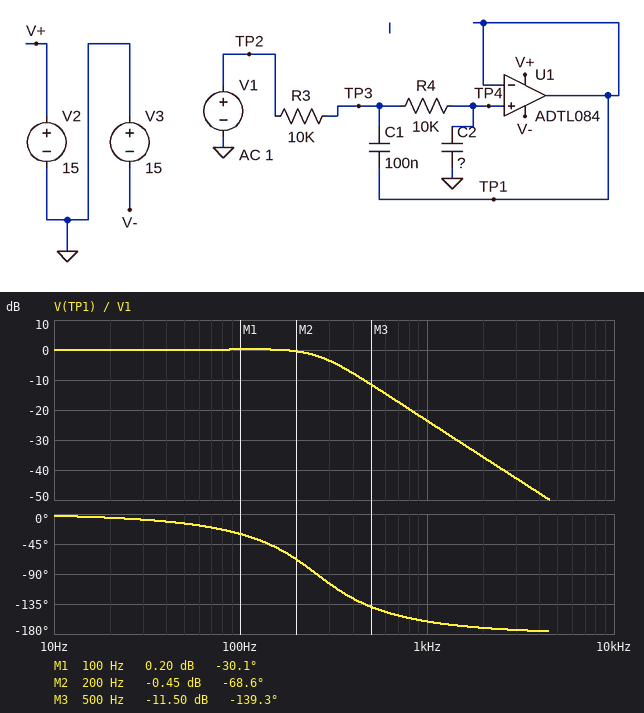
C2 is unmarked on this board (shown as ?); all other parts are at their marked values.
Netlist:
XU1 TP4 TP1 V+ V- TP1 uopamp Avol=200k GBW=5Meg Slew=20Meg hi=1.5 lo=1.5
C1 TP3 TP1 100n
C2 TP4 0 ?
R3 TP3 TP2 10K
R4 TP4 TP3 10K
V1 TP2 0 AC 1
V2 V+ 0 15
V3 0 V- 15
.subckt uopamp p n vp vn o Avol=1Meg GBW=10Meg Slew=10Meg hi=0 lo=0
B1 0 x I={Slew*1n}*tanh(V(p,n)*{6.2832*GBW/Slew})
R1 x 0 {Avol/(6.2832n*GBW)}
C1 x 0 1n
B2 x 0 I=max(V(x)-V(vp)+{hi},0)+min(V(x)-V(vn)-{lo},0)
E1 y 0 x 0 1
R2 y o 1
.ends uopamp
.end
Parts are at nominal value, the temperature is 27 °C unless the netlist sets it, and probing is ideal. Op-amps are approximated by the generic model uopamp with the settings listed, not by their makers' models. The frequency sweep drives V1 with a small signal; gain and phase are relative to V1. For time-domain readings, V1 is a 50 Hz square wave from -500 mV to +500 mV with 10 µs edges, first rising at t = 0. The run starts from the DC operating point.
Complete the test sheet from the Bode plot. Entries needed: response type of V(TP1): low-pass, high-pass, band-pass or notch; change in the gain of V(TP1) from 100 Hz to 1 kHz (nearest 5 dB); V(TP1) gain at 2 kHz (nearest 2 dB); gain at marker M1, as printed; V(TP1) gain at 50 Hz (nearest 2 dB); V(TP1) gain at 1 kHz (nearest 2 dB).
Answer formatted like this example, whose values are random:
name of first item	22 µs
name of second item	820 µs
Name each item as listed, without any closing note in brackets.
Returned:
response type of V(TP1): low-pass, high-pass, band-pass or notch	low-pass
change in the gain of V(TP1) from 100 Hz to 1 kHz	-25 dB
V(TP1) gain at 2 kHz	-36 dB
gain at marker M1, as printed	0.20 dB
V(TP1) gain at 50 Hz	0 dB
V(TP1) gain at 1 kHz	-24 dB
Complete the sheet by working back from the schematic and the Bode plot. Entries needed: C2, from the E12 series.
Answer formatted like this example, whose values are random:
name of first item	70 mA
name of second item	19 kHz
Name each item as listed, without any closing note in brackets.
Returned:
C2, from the E12 series	39 nF
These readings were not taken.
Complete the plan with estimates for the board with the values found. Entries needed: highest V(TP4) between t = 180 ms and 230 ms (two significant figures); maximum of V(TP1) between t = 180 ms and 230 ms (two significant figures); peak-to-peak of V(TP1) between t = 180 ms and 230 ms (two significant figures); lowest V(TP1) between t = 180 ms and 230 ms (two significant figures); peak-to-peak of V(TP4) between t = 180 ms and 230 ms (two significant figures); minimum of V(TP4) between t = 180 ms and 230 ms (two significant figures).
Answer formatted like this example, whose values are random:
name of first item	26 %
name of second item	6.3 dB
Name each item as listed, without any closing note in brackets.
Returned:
highest V(TP4) between t = 180 ms and 230 ms	580 mV
maximum of V(TP1) between t = 180 ms and 230 ms	580 mV
peak-to-peak of V(TP1) between t = 180 ms and 230 ms	1.2 V
lowest V(TP1) between t = 180 ms and 230 ms	-580 mV
peak-to-peak of V(TP4) between t = 180 ms and 230 ms	1.2 V
minimum of V(TP4) between t = 180 ms and 230 ms	-580 mV
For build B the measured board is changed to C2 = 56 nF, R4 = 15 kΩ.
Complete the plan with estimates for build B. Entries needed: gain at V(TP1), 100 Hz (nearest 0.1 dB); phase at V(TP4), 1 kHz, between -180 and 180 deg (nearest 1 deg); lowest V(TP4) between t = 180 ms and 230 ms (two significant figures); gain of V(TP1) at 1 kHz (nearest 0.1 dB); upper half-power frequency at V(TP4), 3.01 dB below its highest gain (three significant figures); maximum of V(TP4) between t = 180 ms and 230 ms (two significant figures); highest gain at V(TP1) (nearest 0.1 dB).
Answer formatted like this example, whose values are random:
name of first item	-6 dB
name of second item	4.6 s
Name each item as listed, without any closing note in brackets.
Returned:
gain at V(TP1), 100 Hz	-0.9 dB
phase at V(TP4), 1 kHz, between -180 and 180 deg	-165 deg
lowest V(TP4) between t = 180 ms and 230 ms	-520 mV
gain of V(TP1) at 1 kHz	-30.5 dB
upper half-power frequency at V(TP4), 3.01 dB below its highest gain	160 Hz
maximum of V(TP4) between t = 180 ms and 230 ms	520 mV
highest gain at V(TP1)	0 dB
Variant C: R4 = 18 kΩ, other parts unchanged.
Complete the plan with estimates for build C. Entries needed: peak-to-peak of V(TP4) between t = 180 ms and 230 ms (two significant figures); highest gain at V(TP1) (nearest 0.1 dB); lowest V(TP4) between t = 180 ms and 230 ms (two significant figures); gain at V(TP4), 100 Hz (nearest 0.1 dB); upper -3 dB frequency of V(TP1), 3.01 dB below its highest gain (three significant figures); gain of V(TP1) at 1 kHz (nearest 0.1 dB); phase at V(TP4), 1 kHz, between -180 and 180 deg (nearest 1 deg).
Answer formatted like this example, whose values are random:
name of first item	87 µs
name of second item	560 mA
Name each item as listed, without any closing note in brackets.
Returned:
peak-to-peak of V(TP4) between t = 180 ms and 230 ms	1.1 V
highest gain at V(TP1)	0.1 dB
lowest V(TP4) between t = 180 ms and 230 ms	-570 mV
gain at V(TP4), 100 Hz	0 dB
upper -3 dB frequency of V(TP1), 3.01 dB below its highest gain	203 Hz
gain of V(TP1) at 1 kHz	-28.8 dB
phase at V(TP4), 1 kHz, between -180 and 180 deg	-166 deg
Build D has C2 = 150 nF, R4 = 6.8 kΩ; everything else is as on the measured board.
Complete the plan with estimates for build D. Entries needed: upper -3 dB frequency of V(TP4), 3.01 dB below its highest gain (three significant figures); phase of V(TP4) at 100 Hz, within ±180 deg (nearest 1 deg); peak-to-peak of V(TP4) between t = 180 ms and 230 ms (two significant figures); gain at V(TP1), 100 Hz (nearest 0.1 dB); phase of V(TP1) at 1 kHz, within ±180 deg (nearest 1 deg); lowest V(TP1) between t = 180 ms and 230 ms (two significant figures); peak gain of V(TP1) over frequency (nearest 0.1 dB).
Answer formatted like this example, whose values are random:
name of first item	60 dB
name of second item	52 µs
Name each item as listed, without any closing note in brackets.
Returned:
upper -3 dB frequency of V(TP4), 3.01 dB below its highest gain	74.7 Hz
phase of V(TP4) at 100 Hz, within ±180 deg	-69 deg
peak-to-peak of V(TP4) between t = 180 ms and 230 ms	980 mV
gain at V(TP1), 100 Hz	-4.6 dB
phase of V(TP1) at 1 kHz, within ±180 deg	-158 deg
lowest V(TP1) between t = 180 ms and 230 ms	-490 mV
peak gain of V(TP1) over frequency	0 dB
